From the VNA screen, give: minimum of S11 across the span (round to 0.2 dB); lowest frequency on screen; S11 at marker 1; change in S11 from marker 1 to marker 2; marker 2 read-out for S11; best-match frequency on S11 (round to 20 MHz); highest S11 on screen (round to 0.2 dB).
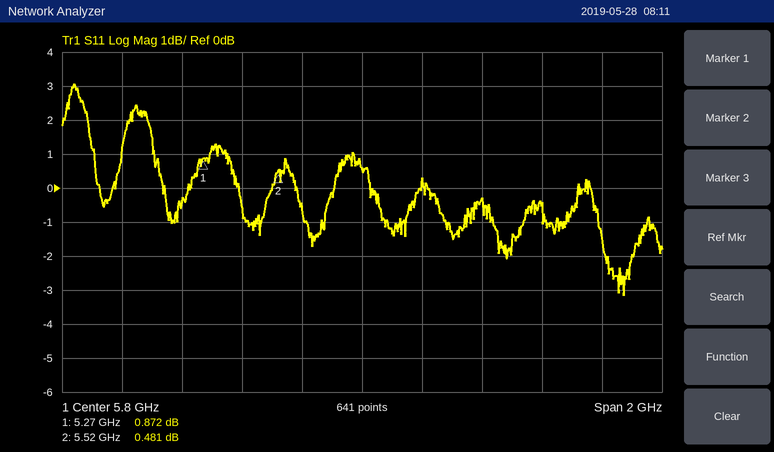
-3.2 dB
4.8 GHz
0.872 dB
-0.391 dB
0.481 dB
6.68 GHz
3.0 dB
